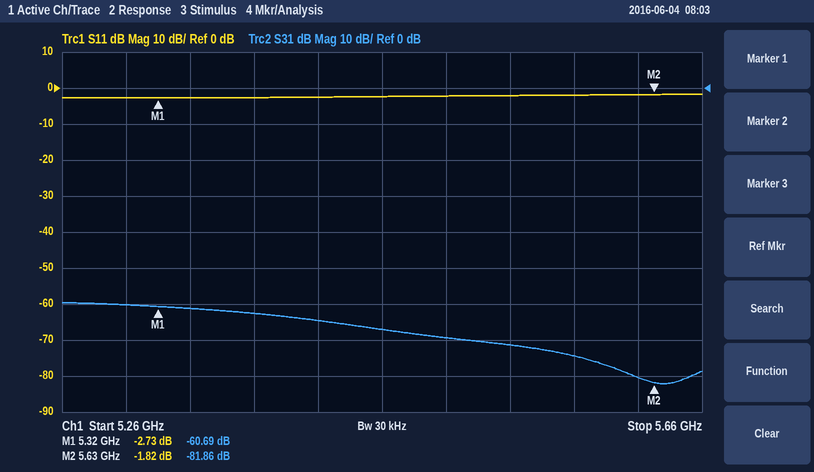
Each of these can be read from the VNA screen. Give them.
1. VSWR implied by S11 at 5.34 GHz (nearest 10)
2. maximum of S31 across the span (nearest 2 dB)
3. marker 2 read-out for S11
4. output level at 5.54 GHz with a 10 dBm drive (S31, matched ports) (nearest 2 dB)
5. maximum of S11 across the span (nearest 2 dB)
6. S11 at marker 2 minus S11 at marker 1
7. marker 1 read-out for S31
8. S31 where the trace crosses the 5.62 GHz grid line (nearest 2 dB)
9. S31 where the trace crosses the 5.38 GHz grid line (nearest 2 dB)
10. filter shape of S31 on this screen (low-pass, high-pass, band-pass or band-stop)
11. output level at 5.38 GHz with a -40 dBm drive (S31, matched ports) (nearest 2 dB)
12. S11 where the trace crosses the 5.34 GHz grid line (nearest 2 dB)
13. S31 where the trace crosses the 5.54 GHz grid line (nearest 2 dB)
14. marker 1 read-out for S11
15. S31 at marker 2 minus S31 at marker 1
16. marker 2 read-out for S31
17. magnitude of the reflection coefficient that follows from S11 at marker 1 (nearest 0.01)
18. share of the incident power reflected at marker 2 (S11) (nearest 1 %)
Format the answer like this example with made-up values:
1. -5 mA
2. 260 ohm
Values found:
1. 10
2. -60 dB
3. -1.82 dB
4. -62 dBm
5. -2 dB
6. 0.91 dB
7. -60.69 dB
8. -80 dB
9. -62 dB
10. low-pass
11. -102 dBm
12. -2 dB
13. -72 dB
14. -2.73 dB
15. -21.17 dB
16. -81.86 dB
17. 0.73
18. 66 %
